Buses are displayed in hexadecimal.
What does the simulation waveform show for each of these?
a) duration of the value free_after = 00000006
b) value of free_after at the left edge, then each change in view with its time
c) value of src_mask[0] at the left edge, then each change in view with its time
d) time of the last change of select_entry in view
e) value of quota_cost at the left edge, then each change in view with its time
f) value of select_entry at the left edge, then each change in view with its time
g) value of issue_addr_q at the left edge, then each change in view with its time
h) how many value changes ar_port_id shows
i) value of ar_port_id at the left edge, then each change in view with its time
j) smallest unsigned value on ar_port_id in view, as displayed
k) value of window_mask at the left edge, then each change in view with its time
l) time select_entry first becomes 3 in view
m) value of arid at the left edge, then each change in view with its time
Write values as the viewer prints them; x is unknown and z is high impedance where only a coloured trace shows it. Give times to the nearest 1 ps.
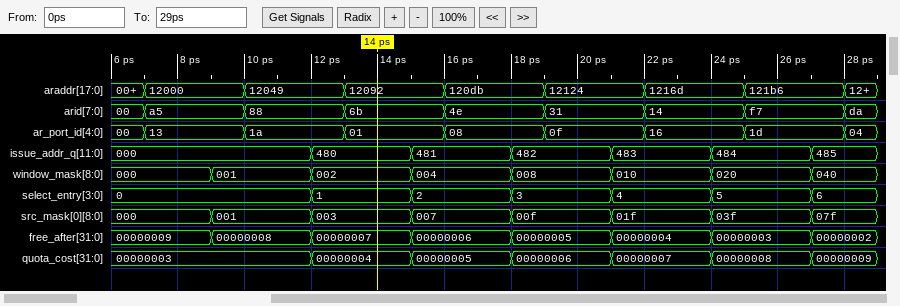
3 ps
00000009, 00000008 at 9 ps, 00000007 at 12 ps, 00000006 at 15 ps, 00000005 at 18 ps, 00000004 at 21 ps, 00000003 at 24 ps, 00000002 at 27 ps
000, 001 at 9 ps, 003 at 12 ps, 007 at 15 ps, 00f at 18 ps, 01f at 21 ps, 03f at 24 ps, 07f at 27 ps
27 ps
00000003, 00000004 at 12 ps, 00000005 at 15 ps, 00000006 at 18 ps, 00000007 at 21 ps, 00000008 at 24 ps, 00000009 at 27 ps
0, 1 at 12 ps, 2 at 15 ps, 3 at 18 ps, 4 at 21 ps, 5 at 24 ps, 6 at 27 ps
000, 480 at 12 ps, 481 at 15 ps, 482 at 18 ps, 483 at 21 ps, 484 at 24 ps, 485 at 27 ps
8
00, 13 at 7 ps, 1a at 10 ps, 01 at 13 ps, 08 at 16 ps, 0f at 19 ps, 16 at 22 ps, 1d at 25 ps, 04 at 28 ps
00
000, 001 at 9 ps, 002 at 12 ps, 004 at 15 ps, 008 at 18 ps, 010 at 21 ps, 020 at 24 ps, 040 at 27 ps
18 ps
00, a5 at 7 ps, 88 at 10 ps, 6b at 13 ps, 4e at 16 ps, 31 at 19 ps, 14 at 22 ps, f7 at 25 ps, da at 28 ps
